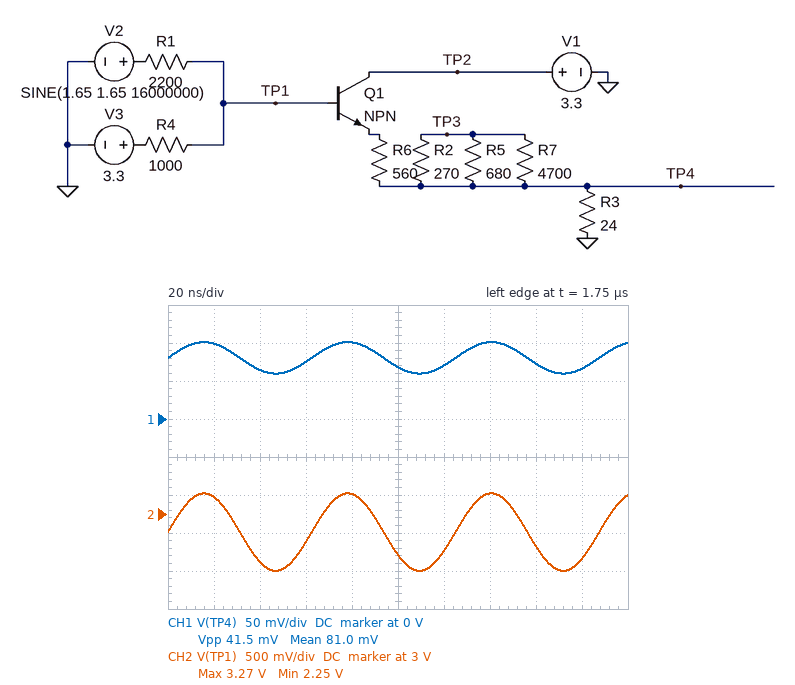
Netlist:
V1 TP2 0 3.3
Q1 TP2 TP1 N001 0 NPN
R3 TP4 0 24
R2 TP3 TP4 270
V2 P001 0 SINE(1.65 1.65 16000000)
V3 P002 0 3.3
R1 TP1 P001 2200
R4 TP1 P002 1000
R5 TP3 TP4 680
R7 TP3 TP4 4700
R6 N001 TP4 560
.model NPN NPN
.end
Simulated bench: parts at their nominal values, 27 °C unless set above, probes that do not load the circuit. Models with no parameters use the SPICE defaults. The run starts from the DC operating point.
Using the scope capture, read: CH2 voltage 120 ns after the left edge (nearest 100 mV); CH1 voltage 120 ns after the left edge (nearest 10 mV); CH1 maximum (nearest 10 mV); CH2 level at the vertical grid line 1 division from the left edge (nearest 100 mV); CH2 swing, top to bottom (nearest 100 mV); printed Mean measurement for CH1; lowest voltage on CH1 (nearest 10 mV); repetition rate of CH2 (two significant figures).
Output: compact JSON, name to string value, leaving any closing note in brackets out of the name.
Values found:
{"CH2 voltage 120 ns after the left edge": "2.5 V", "CH1 voltage 120 ns after the left edge": "70 mV", "CH1 maximum": "100 mV", "CH2 level at the vertical grid line 1 division from the left edge": "3.2 V", "CH2 swing, top to bottom": "1.0 V", "printed Mean measurement for CH1": "81.0 mV", "lowest voltage on CH1": "60 mV", "repetition rate of CH2": "16 MHz"}
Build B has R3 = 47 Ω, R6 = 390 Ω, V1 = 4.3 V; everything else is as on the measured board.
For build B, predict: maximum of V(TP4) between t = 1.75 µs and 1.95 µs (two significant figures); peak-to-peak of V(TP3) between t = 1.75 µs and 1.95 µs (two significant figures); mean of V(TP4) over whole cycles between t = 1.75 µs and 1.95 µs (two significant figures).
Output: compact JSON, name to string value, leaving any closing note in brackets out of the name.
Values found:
{"maximum of V(TP4) between t = 1.75 µs and 1.95 µs": "260 mV", "peak-to-peak of V(TP3) between t = 1.75 µs and 1.95 µs": "110 mV", "mean of V(TP4) over whole cycles between t = 1.75 µs and 1.95 µs": "210 mV"}
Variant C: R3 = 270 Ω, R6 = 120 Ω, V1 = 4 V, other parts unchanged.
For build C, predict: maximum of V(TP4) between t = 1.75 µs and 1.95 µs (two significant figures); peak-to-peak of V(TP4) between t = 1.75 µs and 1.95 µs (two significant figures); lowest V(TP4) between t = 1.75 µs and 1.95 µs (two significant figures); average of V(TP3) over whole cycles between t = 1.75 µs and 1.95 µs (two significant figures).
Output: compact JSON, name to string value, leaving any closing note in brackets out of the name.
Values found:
{"maximum of V(TP4) between t = 1.75 µs and 1.95 µs": "1.7 V", "peak-to-peak of V(TP4) between t = 1.75 µs and 1.95 µs": "690 mV", "lowest V(TP4) between t = 1.75 µs and 1.95 µs": "990 mV", "average of V(TP3) over whole cycles between t = 1.75 µs and 1.95 µs": "1.3 V"}
